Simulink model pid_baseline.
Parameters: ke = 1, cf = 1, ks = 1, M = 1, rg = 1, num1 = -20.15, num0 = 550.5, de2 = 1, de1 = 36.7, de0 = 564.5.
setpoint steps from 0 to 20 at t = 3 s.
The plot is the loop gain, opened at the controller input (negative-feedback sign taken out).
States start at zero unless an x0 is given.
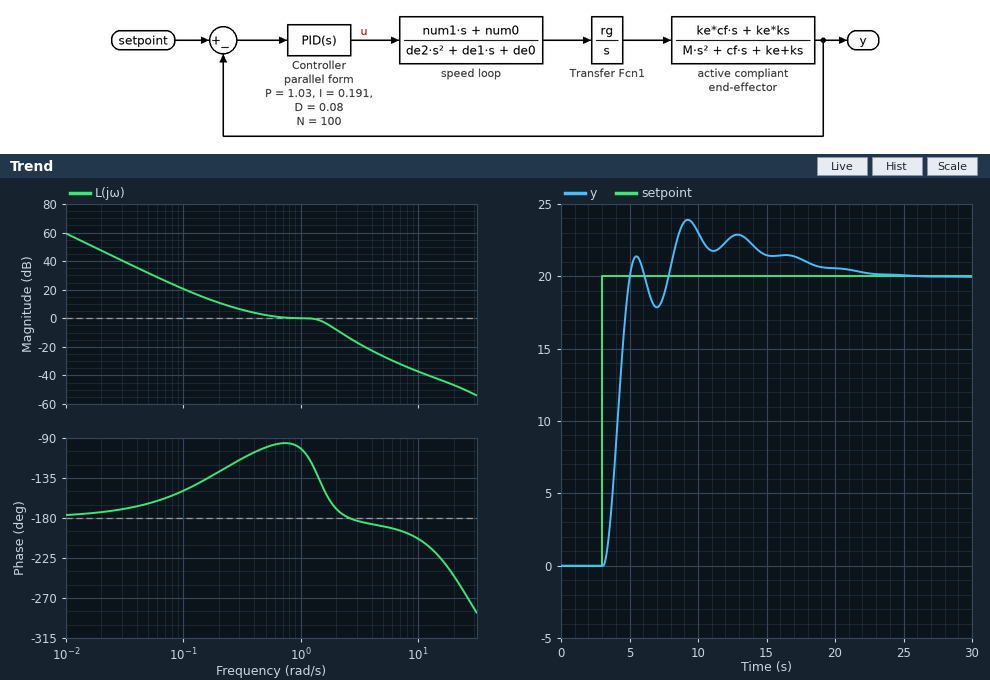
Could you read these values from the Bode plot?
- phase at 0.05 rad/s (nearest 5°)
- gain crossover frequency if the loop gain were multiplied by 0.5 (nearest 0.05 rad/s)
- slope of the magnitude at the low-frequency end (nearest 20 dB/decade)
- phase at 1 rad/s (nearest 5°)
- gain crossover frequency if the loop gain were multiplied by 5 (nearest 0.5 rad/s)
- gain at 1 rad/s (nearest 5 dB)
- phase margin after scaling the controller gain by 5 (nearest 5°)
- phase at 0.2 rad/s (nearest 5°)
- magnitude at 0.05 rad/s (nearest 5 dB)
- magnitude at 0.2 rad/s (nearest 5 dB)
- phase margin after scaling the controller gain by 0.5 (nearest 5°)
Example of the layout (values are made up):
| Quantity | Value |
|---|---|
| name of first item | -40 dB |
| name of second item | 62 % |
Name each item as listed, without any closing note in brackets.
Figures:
| Quantity | Value |
|---|---|
| phase at 0.05 rad/s | -165° |
| gain crossover frequency if the loop gain were multiplied by 0.5 | 0.30 rad/s |
| slope of the magnitude at the low-frequency end | -40 dB/decade |
| phase at 1 rad/s | -100° |
| gain crossover frequency if the loop gain were multiplied by 5 | 2.5 rad/s |
| gain at 1 rad/s | 0 dB |
| phase margin after scaling the controller gain by 5 | 0° |
| phase at 0.2 rad/s | -130° |
| magnitude at 0.05 rad/s | 30 dB |
| magnitude at 0.2 rad/s | 10 dB |
| phase margin after scaling the controller gain by 0.5 | 65° |
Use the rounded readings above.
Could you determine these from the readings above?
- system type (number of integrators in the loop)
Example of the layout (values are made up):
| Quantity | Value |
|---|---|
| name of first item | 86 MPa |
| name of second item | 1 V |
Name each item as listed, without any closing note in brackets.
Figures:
| Quantity | Value |
|---|---|
| system type | 2 |
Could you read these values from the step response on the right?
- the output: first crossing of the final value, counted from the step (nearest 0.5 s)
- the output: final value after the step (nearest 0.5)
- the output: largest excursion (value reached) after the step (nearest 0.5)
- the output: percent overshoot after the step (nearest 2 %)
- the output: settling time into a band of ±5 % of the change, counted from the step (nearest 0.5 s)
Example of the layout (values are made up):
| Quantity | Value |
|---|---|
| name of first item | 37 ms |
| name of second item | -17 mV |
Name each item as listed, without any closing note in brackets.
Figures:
| Quantity | Value |
|---|---|
| the output: first crossing of the final value, counted from the step | 2.0 s |
| the output: final value after the step | 20.0 |
| the output: largest excursion (value reached) after the step | 24.0 |
| the output: percent overshoot after the step | 20 % |
| the output: settling time into a band of ±5 % of the change, counted from the step | 15.0 s |
